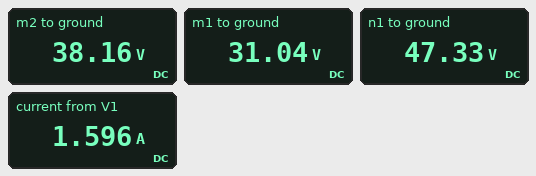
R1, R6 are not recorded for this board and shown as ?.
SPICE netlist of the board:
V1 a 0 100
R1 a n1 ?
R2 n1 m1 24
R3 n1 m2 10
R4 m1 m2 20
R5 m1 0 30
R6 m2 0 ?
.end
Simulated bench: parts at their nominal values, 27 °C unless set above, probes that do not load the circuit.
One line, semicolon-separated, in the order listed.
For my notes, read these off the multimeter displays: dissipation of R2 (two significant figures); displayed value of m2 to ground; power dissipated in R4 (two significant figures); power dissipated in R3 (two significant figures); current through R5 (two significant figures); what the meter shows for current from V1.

11 W; 38.16 V; 2.5 W; 8.4 W; 1.0 A; 1.596 A
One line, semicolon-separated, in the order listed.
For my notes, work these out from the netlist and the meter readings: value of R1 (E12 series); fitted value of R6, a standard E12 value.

33 Ω; 68 Ω
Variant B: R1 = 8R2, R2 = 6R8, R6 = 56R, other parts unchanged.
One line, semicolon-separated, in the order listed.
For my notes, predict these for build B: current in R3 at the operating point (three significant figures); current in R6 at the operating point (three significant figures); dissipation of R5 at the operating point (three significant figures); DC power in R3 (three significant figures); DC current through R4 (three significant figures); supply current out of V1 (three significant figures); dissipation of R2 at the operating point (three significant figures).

1.19 A; 1.11 A; 124 W; 14.1 W; 72.6 mA; 3.14 A; 26.1 W
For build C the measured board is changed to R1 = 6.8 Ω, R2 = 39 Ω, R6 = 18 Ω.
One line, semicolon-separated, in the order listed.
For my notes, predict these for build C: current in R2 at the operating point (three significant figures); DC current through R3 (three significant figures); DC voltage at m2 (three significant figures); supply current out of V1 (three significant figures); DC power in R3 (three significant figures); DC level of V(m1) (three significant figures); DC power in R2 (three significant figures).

920 mA; 2.88 A; 45.4 V; 3.80 A; 82.8 W; 38.3 V; 33.0 W
